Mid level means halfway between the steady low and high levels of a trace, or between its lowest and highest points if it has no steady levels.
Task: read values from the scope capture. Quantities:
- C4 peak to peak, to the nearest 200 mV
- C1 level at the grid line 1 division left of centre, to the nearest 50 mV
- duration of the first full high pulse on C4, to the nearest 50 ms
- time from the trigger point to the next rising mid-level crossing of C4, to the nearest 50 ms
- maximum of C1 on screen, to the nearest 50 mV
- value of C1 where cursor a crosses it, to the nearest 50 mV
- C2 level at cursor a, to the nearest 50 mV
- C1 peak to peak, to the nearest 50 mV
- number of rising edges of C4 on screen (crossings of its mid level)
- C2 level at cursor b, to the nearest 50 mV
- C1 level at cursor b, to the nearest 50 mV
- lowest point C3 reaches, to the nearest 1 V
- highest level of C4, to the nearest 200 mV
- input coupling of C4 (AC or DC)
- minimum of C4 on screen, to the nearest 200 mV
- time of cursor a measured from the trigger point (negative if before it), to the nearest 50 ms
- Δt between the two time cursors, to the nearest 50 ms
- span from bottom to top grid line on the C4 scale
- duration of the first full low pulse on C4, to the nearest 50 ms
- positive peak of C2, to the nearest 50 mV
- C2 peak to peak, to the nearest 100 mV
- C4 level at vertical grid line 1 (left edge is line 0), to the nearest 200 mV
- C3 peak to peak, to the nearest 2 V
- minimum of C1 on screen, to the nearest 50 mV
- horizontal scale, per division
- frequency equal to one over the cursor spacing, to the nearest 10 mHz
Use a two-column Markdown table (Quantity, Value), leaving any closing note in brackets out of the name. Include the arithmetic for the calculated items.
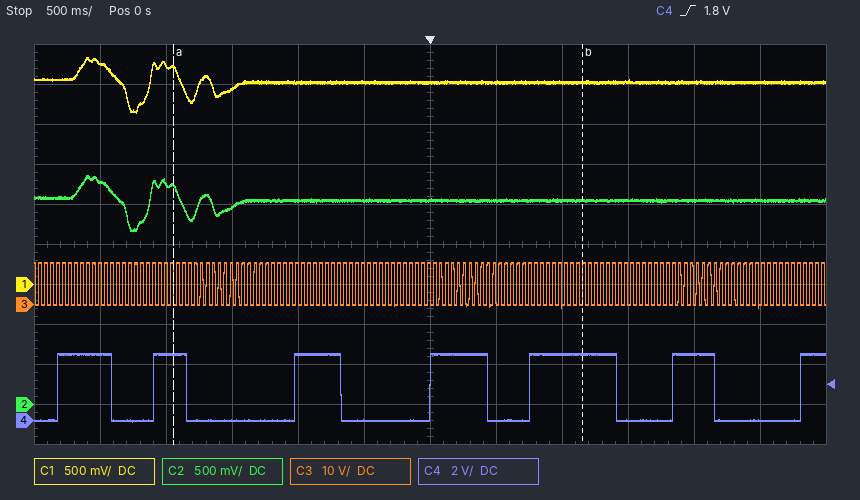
| Quantity | Value |
|---|---|
| C4 peak to peak, to the nearest 200 mV | 3.4 V − (0.0 V) = 3.4 V |
| C1 level at the grid line 1 division left of centre, to the nearest 50 mV | 2.55 V |
| duration of the first full high pulse on C4, to the nearest 50 ms | 400 ms |
| time from the trigger point to the next rising mid-level crossing of C4, to the nearest 50 ms | 750 ms |
| maximum of C1 on screen, to the nearest 50 mV | 2.85 V |
| value of C1 where cursor a crosses it, to the nearest 50 mV | 2.70 V |
| C2 level at cursor a, to the nearest 50 mV | 2.70 V |
| C1 peak to peak, to the nearest 50 mV | 2.85 V − (2.15 V) = 700 mV |
| number of rising edges of C4 on screen | 7 |
| C2 level at cursor b, to the nearest 50 mV | 2.55 V |
| C1 level at cursor b, to the nearest 50 mV | 2.55 V |
| lowest point C3 reaches, to the nearest 1 V | -1 V |
| highest level of C4, to the nearest 200 mV | 3.4 V |
| input coupling of C4 | DC |
| minimum of C4 on screen, to the nearest 200 mV | 0.0 V |
| time of cursor a measured from the trigger point (negative if before it), to the nearest 50 ms | -1.95 s |
| Δt between the two time cursors, to the nearest 50 ms | 3.10 s |
| span from bottom to top grid line on the C4 scale | 20 V |
| duration of the first full low pulse on C4, to the nearest 50 ms | 300 ms |
| positive peak of C2, to the nearest 50 mV | 2.85 V |
| C2 peak to peak, to the nearest 100 mV | 700 mV |
| C4 level at vertical grid line 1 (left edge is line 0), to the nearest 200 mV | 3.4 V |
| C3 peak to peak, to the nearest 2 V | 12 V |
| minimum of C1 on screen, to the nearest 50 mV | 2.15 V |
| horizontal scale, per division | 500 ms |
| frequency equal to one over the cursor spacing, to the nearest 10 mHz | 1 / 3.10 s ≈ 320 mHz |
